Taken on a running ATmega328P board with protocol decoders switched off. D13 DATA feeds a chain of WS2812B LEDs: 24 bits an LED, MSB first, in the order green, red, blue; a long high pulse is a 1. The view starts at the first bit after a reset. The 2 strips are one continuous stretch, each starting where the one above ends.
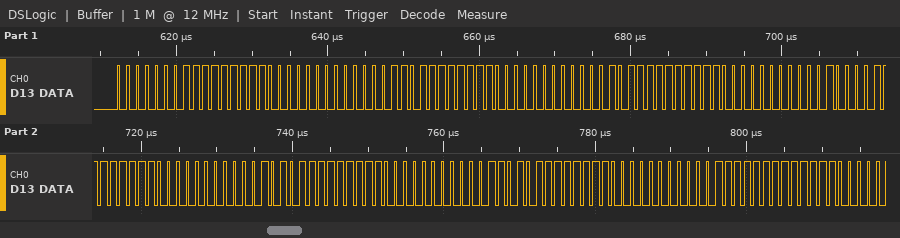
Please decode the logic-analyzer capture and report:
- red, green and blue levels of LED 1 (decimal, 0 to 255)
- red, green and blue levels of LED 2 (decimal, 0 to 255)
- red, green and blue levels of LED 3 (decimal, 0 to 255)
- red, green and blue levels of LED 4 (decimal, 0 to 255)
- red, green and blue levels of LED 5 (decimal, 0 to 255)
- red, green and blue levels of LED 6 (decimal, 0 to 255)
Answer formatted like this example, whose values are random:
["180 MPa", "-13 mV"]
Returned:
["255, 1, 0", "255, 6, 0", "255, 11, 0", "255, 16, 0", "255, 21, 0", "255, 26, 0"]
